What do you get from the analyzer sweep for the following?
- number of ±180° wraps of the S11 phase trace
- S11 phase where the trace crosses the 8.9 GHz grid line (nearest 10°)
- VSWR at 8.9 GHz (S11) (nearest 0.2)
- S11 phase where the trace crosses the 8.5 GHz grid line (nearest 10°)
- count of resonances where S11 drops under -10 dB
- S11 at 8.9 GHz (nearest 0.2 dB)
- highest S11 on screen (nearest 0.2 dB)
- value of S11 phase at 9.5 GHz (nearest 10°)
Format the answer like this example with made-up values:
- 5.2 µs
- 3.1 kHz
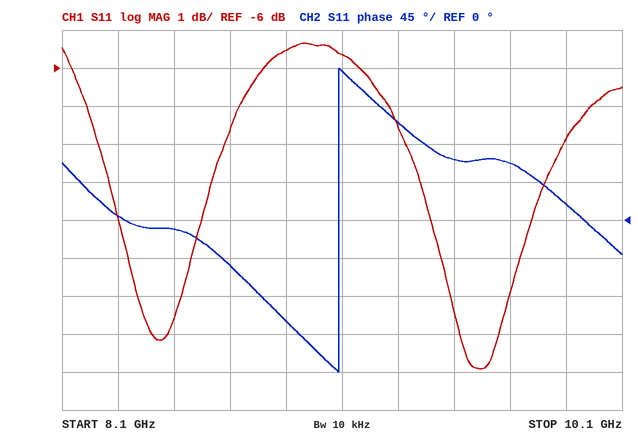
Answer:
- 1
- -120°
- 3.2
- -10°
- 2
- -5.6 dB
- -5.4 dB
- 70°
